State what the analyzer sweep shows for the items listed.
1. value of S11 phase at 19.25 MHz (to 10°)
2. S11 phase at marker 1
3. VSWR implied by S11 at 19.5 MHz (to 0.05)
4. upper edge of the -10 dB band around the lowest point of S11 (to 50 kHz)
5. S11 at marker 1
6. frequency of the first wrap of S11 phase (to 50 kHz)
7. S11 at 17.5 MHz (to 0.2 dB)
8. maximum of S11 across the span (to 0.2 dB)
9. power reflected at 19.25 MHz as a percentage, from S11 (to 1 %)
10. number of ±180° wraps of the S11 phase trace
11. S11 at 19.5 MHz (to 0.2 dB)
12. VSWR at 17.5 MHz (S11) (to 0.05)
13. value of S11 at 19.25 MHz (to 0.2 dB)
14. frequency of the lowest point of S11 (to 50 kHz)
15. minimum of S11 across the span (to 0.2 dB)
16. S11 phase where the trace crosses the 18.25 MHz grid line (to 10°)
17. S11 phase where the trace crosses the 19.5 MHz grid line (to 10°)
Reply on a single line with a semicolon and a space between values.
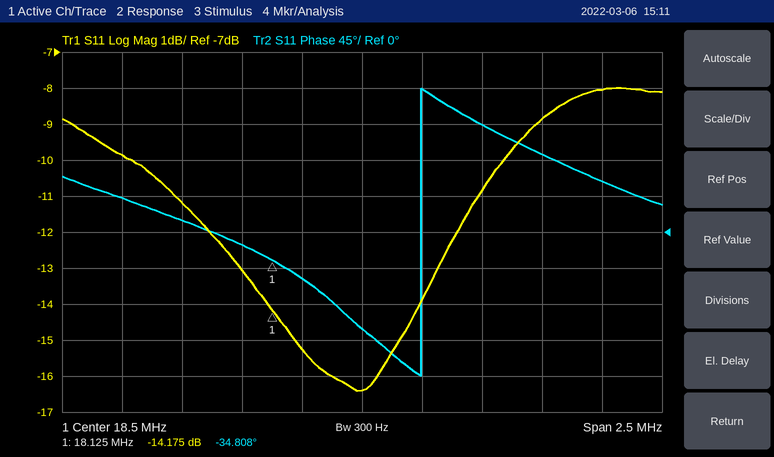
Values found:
100°; -34.808°; 2.30; 19.10 MHz; -14.175 dB; 18.75 MHz; -9.8 dB; -8.0 dB; 13 %; 1; -8.0 dB; 1.95; -8.8 dB; 18.50 MHz; -16.4 dB; -60°; 60°
